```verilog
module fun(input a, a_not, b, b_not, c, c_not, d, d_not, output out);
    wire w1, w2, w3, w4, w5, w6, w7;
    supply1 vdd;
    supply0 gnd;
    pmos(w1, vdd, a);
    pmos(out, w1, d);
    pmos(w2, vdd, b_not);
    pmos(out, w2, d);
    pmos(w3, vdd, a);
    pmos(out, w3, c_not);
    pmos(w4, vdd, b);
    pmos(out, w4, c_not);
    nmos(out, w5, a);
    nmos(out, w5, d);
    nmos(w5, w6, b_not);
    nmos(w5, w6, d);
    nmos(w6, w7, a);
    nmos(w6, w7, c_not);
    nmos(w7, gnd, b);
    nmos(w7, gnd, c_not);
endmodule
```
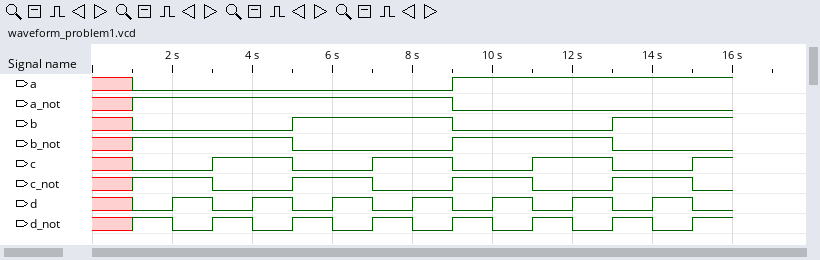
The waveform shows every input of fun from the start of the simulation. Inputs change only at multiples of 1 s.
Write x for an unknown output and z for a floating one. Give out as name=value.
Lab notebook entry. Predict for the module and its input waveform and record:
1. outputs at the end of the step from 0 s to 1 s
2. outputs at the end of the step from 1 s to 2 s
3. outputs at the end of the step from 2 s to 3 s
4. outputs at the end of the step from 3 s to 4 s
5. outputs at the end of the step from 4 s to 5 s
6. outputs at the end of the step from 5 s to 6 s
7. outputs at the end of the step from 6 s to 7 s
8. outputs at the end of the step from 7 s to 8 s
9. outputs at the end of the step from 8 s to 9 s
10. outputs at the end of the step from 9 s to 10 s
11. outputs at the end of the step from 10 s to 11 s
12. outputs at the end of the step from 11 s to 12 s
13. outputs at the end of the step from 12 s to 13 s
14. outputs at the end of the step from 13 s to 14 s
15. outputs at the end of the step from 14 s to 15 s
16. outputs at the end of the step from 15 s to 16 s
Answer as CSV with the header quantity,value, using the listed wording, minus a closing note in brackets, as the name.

quantity,value
outputs at the end of the step from 0 s to 1 s,out=x
outputs at the end of the step from 1 s to 2 s,out=1
outputs at the end of the step from 2 s to 3 s,out=0
outputs at the end of the step from 3 s to 4 s,out=1
outputs at the end of the step from 4 s to 5 s,out=1
outputs at the end of the step from 5 s to 6 s,out=1
outputs at the end of the step from 6 s to 7 s,out=0
outputs at the end of the step from 7 s to 8 s,out=1
outputs at the end of the step from 8 s to 9 s,out=1
outputs at the end of the step from 9 s to 10 s,out=0
outputs at the end of the step from 10 s to 11 s,out=0
outputs at the end of the step from 11 s to 12 s,out=1
outputs at the end of the step from 12 s to 13 s,out=1
outputs at the end of the step from 13 s to 14 s,out=1
outputs at the end of the step from 14 s to 15 s,out=0
outputs at the end of the step from 15 s to 16 s,out=1
